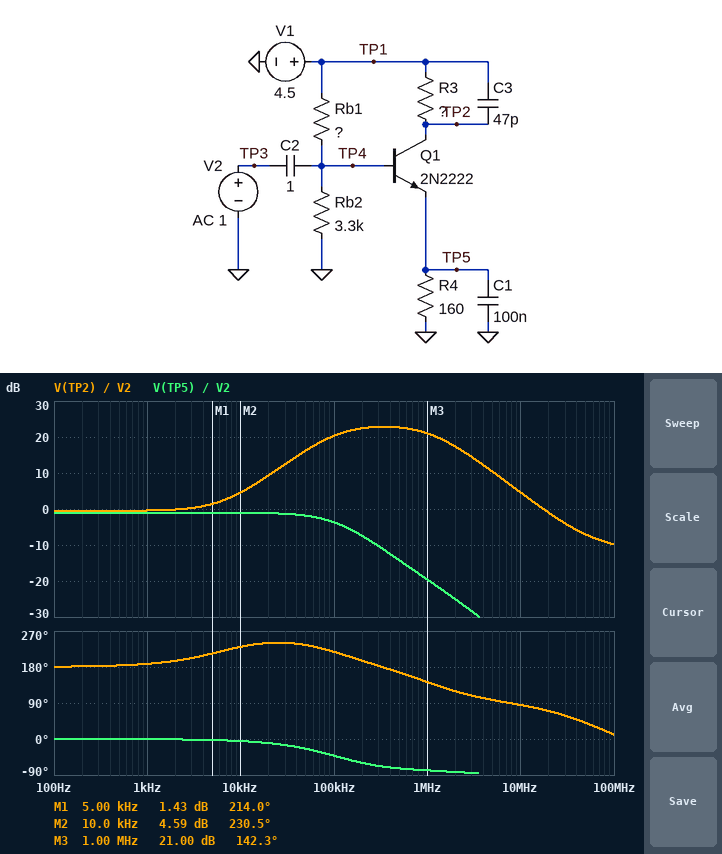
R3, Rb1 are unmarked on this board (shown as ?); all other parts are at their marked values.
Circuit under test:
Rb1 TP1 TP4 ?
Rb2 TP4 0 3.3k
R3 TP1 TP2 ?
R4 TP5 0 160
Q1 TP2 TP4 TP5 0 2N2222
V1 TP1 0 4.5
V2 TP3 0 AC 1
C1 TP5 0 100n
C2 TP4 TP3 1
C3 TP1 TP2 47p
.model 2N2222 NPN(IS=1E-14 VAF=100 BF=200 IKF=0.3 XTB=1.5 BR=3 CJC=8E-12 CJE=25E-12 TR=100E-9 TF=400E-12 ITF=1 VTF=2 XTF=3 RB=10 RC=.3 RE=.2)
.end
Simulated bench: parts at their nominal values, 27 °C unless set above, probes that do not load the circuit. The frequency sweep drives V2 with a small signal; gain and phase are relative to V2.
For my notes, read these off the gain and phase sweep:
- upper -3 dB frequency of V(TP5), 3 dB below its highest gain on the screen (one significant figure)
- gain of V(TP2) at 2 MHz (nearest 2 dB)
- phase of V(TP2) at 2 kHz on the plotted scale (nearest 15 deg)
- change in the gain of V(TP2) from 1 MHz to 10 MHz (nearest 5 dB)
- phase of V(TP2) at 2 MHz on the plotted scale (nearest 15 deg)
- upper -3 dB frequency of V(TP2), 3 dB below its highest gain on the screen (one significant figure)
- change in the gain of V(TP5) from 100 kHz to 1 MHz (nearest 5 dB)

100 kHz
18 dB
195 deg
-15 dB
120 deg
1 MHz
-15 dB
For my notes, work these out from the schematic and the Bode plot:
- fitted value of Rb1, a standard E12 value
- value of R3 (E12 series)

4.7 kΩ
560 Ω
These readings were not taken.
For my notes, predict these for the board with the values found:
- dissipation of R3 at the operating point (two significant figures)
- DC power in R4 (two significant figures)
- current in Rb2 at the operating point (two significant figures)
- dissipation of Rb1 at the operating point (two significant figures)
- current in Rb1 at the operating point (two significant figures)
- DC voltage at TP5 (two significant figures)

21 mW
6.1 mW
510 µA
1.7 mW
600 µA
990 mV
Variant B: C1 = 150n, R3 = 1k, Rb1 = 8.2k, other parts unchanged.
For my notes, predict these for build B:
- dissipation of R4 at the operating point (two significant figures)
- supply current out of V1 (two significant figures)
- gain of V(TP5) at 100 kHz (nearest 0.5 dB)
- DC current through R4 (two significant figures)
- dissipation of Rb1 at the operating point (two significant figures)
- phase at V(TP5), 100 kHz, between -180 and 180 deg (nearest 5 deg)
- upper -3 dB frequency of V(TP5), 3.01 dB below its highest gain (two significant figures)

2.0 mW
3.9 mA
-2.0 dB
3.5 mA
1.3 mW
-35 deg
140 kHz
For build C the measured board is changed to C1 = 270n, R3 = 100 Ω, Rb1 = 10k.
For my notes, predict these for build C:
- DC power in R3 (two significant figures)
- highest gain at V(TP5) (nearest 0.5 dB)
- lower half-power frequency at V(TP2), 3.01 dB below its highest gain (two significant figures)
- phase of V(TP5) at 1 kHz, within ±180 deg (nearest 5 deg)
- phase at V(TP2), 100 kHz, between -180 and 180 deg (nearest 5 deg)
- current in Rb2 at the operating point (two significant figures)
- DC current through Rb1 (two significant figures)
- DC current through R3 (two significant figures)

640 µW
-0.5 dB
59 kHz
0 deg
-150 deg
330 µA
340 µA
2.5 mA
